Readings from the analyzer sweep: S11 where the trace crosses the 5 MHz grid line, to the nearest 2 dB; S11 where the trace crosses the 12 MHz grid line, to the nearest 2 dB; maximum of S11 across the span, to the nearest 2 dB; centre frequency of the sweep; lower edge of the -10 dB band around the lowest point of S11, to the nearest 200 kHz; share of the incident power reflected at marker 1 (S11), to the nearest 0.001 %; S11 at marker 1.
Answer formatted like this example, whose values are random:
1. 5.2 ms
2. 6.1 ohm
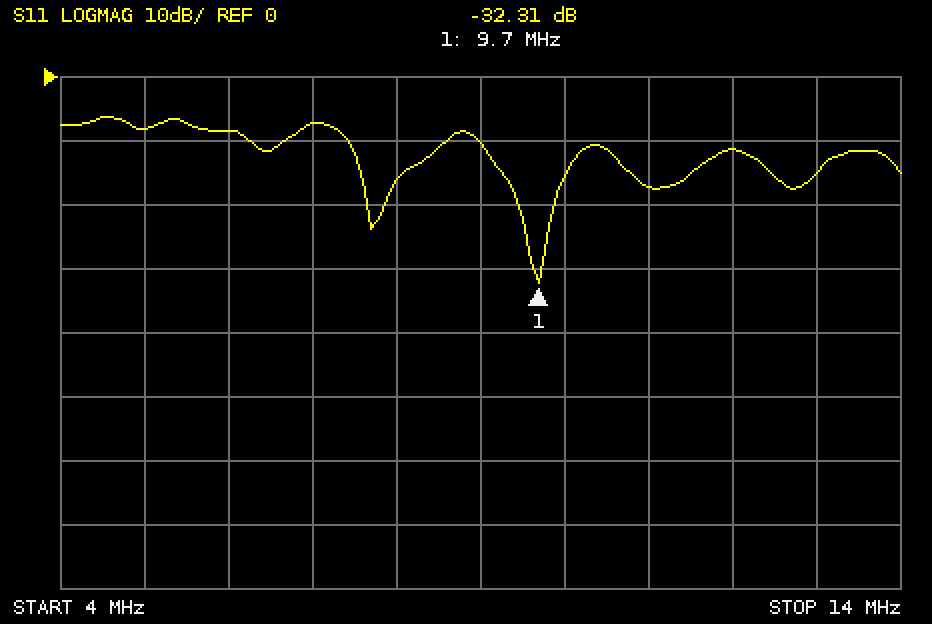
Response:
1. -8 dB
2. -12 dB
3. -6 dB
4. 9 MHz
5. 9.0 MHz
6. 0.059 %
7. -32.31 dB
